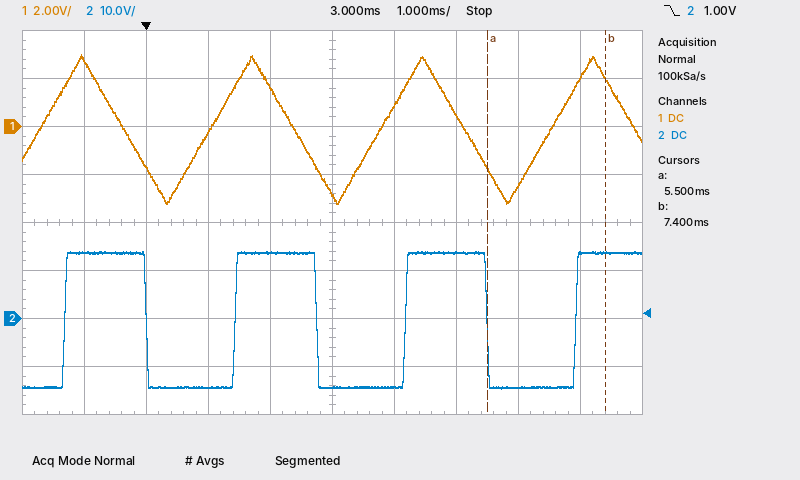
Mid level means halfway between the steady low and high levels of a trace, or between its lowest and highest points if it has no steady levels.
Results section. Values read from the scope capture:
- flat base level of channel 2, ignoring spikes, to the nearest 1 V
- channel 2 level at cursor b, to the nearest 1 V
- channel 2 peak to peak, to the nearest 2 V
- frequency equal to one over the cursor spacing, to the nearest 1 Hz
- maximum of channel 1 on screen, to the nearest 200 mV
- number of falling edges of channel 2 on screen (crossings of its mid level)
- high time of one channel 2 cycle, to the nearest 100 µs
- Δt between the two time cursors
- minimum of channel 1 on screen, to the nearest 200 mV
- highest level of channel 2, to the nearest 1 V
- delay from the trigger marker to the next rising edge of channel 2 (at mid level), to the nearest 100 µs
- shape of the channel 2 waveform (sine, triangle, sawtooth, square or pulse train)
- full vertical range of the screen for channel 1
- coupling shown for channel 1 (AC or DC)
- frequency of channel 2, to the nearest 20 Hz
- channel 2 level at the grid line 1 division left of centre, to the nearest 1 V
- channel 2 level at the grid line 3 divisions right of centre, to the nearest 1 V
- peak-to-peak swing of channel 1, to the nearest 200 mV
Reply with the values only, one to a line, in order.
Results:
-14 V
14 V
28 V
526 Hz
3.0 V
3
1.3 ms
1.9 ms
-3.2 V
14 V
1.4 ms
square
16 V
DC
360 Hz
14 V
-14 V
6.2 V
